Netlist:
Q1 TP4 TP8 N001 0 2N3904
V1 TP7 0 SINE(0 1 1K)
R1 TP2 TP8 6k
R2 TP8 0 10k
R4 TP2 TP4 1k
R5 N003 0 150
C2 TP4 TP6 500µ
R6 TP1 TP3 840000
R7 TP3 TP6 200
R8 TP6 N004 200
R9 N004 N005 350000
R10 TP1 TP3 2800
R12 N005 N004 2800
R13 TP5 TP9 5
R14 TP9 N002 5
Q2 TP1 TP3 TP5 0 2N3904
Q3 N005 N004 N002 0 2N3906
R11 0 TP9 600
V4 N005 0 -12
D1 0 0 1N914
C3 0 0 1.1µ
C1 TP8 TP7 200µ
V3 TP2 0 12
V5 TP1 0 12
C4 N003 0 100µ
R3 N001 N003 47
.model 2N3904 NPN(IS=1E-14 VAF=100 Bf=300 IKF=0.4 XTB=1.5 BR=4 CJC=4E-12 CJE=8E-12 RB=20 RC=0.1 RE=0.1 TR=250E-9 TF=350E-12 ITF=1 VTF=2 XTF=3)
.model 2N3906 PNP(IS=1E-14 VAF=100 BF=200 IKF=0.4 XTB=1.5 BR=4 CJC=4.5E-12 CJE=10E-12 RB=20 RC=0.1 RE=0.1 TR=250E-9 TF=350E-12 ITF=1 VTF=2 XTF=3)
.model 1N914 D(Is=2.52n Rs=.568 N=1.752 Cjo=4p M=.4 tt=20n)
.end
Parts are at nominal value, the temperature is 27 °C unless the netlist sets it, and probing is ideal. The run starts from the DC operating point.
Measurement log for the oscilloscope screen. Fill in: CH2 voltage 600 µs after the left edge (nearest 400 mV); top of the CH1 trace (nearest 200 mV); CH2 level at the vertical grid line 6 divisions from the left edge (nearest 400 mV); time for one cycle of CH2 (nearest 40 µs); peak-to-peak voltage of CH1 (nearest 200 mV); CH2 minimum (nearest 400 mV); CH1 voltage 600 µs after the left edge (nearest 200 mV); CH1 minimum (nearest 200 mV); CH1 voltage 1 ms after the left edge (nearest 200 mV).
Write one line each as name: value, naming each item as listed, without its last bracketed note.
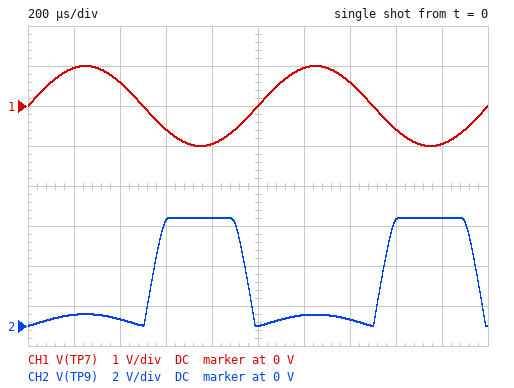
CH2 voltage 600 µs after the left edge: 5.2 V
top of the CH1 trace: 1.0 V
CH2 level at the vertical grid line 6 divisions from the left edge: 400 mV
time for one cycle of CH2: 1.00 ms
peak-to-peak voltage of CH1: 2.0 V
CH2 minimum: 0 V
CH1 voltage 600 µs after the left edge: -600 mV
CH1 minimum: -1.0 V
CH1 voltage 1 ms after the left edge: 0 V
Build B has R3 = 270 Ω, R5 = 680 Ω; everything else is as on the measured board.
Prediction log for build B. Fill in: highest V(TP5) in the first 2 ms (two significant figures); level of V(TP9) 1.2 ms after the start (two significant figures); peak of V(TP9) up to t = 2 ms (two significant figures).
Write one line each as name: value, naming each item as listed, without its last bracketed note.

highest V(TP5) in the first 2 ms: 2.0 V
level of V(TP9) 1.2 ms after the start: 720 mV
peak of V(TP9) up to t = 2 ms: 1.9 V
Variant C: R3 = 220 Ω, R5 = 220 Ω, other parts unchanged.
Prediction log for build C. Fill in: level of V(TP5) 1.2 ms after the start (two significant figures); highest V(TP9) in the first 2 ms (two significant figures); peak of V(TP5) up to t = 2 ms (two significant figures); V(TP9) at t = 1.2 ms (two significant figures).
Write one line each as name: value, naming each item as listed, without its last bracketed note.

level of V(TP5) 1.2 ms after the start: 810 mV
highest V(TP9) in the first 2 ms: 2.0 V
peak of V(TP5) up to t = 2 ms: 2.1 V
V(TP9) at t = 1.2 ms: 730 mV
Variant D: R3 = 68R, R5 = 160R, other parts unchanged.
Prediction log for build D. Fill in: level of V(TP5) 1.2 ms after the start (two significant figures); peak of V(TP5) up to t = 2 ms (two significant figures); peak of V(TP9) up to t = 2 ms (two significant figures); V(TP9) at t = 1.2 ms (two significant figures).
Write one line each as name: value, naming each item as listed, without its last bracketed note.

level of V(TP5) 1.2 ms after the start: 680 mV
peak of V(TP5) up to t = 2 ms: 5.4 V
peak of V(TP9) up to t = 2 ms: 5.3 V
V(TP9) at t = 1.2 ms: 600 mV
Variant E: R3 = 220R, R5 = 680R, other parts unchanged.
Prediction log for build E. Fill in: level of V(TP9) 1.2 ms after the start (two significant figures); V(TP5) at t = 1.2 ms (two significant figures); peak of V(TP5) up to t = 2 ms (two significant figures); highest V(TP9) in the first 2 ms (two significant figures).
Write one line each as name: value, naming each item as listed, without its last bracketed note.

level of V(TP9) 1.2 ms after the start: 710 mV
V(TP5) at t = 1.2 ms: 780 mV
peak of V(TP5) up to t = 2 ms: 2.4 V
highest V(TP9) in the first 2 ms: 2.3 V
